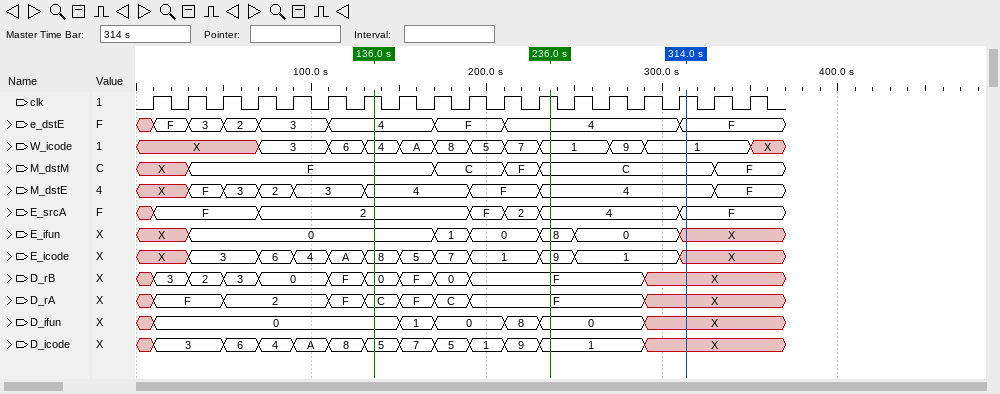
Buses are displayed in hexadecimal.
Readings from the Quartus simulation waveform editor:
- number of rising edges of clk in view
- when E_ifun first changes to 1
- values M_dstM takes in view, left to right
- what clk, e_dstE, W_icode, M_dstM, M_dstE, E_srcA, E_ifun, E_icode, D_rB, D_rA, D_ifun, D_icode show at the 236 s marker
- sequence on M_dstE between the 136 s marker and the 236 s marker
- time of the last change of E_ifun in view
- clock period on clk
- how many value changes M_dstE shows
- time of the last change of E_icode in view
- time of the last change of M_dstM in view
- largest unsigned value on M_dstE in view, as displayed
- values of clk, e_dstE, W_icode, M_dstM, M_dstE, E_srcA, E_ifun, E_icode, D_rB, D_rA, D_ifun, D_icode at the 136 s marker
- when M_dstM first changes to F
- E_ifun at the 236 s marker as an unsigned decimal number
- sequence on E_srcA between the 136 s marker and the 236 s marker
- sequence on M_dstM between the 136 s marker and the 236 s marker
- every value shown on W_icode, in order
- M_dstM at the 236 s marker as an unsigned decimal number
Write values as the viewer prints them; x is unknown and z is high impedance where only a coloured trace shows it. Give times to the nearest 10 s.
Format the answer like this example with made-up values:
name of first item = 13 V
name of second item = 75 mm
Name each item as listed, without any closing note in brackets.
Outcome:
number of rising edges of clk in view = 18
when E_ifun first changes to 1 = 170 s
values M_dstM takes in view, left to right = X, F, C, F, C, F
what clk, e_dstE, W_icode, M_dstM, M_dstE, E_srcA, E_ifun, E_icode, D_rB, D_rA, D_ifun, D_icode show at the 236 s marker = clk=1, e_dstE=4, W_icode=1, M_dstM=C, M_dstE=4, E_srcA=4, E_ifun=8, E_icode=9, D_rB=F, D_rA=F, D_ifun=0, D_icode=1
sequence on M_dstE between the 136 s marker and the 236 s marker = 4, F, 4
time of the last change of E_ifun in view = 310 s
clock period on clk = 20 s
how many value changes M_dstE shows = 8
time of the last change of E_icode in view = 310 s
time of the last change of M_dstM in view = 330 s
largest unsigned value on M_dstE in view, as displayed = F
values of clk, e_dstE, W_icode, M_dstM, M_dstE, E_srcA, E_ifun, E_icode, D_rB, D_rA, D_ifun, D_icode at the 136 s marker = clk=1, e_dstE=4, W_icode=4, M_dstM=F, M_dstE=4, E_srcA=2, E_ifun=0, E_icode=8, D_rB=0, D_rA=C, D_ifun=0, D_icode=5
when M_dstM first changes to F = 30 s
E_ifun at the 236 s marker as an unsigned decimal number = 8
sequence on E_srcA between the 136 s marker and the 236 s marker = 2, F, 2, 4
sequence on M_dstM between the 136 s marker and the 236 s marker = F, C, F, C
every value shown on W_icode, in order = X, 3, 6, 4, A, 8, 5, 7, 1, 9, 1, X
M_dstM at the 236 s marker as an unsigned decimal number = 12
